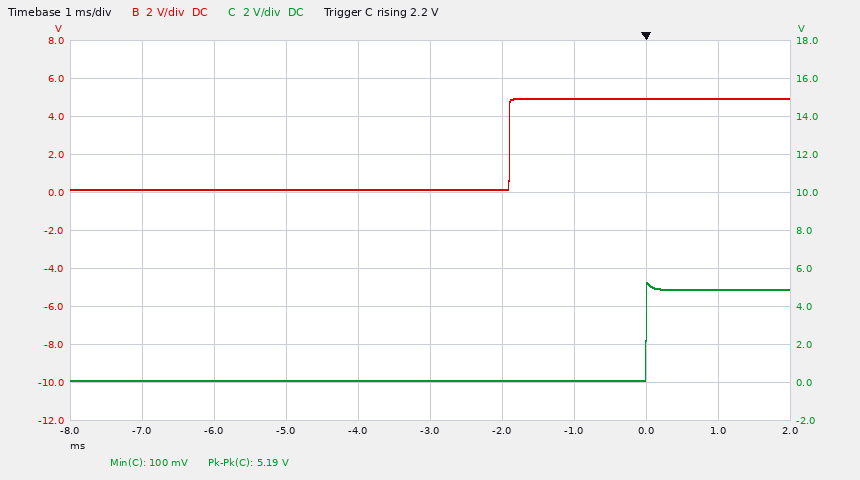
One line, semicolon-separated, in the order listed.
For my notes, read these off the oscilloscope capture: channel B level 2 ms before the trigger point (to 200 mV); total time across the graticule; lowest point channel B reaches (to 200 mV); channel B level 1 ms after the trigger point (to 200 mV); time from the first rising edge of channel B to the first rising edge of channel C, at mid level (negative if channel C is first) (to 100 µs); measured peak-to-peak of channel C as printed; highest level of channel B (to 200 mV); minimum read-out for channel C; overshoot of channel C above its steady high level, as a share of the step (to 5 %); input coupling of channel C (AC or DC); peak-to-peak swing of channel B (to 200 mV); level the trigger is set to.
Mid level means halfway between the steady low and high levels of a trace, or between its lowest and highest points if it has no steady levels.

200 mV; 10 ms; 200 mV; 5.0 V; +1.9 ms; 5.19 V; 5.0 V; 100 mV; 10 %; DC; 4.8 V; 2.2 V
